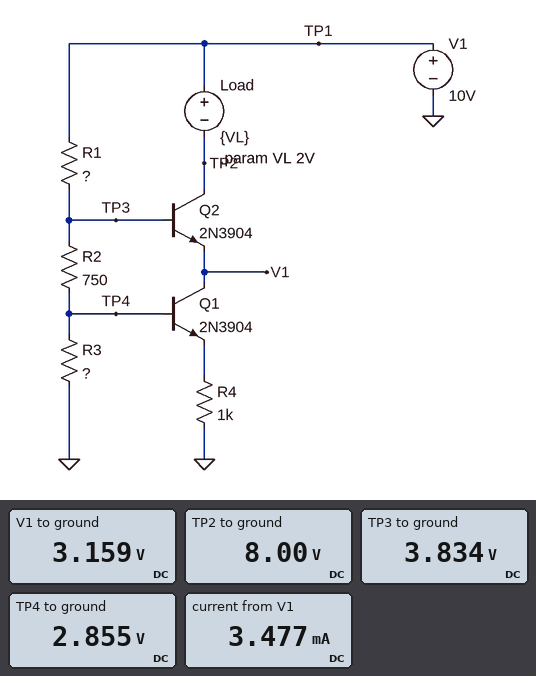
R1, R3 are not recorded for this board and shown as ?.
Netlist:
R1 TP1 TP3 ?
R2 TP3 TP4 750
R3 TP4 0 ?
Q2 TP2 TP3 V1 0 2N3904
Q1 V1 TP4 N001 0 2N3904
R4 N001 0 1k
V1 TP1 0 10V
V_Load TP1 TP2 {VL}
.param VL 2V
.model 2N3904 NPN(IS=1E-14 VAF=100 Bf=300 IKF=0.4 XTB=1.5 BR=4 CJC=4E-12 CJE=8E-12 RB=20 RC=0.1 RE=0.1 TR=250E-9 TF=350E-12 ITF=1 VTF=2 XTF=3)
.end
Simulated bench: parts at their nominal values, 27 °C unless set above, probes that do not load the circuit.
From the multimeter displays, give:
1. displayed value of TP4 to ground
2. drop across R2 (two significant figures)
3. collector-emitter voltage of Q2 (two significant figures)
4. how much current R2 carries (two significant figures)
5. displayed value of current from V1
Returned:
2.855 V
980 mV
4.8 V
1.3 mA
3.477 mA
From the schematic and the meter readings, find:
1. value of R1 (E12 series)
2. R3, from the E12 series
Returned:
4.7 kΩ
2.2 kΩ
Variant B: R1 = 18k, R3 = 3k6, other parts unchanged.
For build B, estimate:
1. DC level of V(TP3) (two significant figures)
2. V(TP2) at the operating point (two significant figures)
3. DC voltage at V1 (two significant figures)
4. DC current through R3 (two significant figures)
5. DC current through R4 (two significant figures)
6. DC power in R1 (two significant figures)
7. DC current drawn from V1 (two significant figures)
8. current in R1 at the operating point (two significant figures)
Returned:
1.9 V
8.0 V
1.3 V
440 µA
940 µA
3.6 mW
1.4 mA
450 µA
